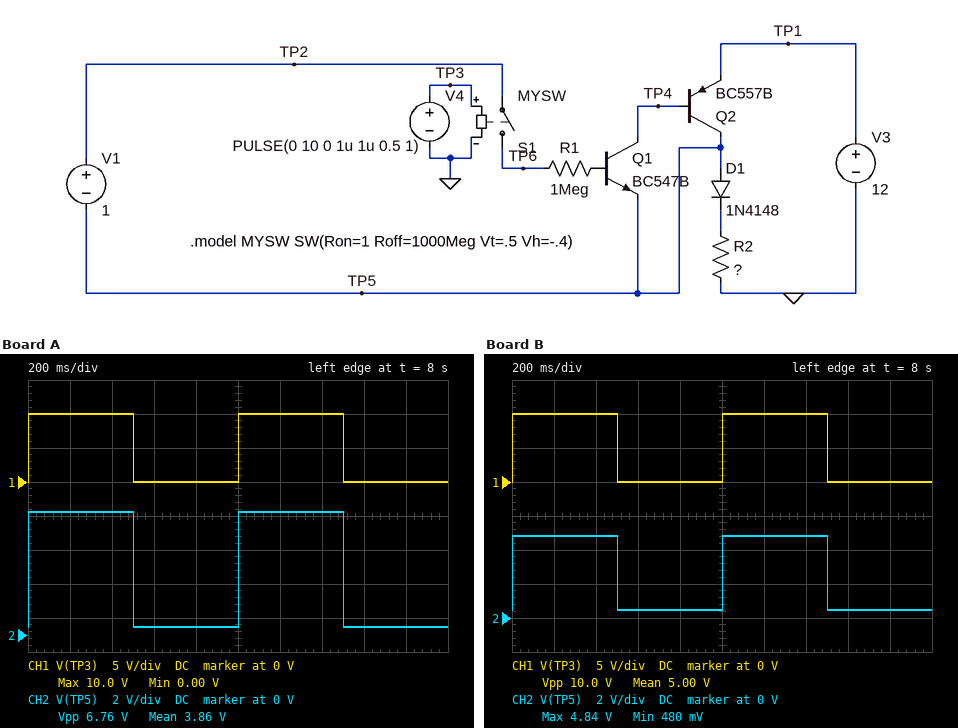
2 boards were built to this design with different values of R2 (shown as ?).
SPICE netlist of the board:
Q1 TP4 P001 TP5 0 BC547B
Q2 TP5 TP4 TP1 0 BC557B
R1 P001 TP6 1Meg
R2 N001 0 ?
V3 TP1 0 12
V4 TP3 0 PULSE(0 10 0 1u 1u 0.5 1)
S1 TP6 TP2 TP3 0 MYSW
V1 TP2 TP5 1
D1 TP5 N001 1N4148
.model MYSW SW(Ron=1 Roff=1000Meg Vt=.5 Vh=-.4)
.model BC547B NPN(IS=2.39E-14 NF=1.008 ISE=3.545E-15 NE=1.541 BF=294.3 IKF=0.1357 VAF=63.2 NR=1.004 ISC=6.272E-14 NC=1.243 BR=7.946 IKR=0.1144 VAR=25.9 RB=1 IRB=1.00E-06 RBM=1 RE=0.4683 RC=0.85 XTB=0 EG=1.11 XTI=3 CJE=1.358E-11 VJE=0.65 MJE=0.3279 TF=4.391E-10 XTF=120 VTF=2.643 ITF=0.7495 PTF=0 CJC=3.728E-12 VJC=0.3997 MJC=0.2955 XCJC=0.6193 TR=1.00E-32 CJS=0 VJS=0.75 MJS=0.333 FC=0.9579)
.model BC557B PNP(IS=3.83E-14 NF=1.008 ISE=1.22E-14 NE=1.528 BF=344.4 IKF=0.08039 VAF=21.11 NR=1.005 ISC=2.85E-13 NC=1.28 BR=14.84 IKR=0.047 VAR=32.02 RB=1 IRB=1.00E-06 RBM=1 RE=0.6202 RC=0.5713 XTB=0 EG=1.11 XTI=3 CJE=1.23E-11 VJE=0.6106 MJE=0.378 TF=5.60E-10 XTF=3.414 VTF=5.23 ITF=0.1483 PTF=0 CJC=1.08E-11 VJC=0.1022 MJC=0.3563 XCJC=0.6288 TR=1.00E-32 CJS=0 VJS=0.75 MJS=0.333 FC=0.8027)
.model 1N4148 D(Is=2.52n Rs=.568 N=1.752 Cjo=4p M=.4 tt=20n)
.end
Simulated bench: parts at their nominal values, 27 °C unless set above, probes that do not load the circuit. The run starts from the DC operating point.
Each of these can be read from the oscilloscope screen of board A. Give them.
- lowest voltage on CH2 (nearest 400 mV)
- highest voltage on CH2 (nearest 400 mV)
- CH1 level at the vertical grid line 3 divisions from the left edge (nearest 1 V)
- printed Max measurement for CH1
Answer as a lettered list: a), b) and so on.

a) 400 mV
b) 7.2 V
c) 0 V
d) 10.0 V
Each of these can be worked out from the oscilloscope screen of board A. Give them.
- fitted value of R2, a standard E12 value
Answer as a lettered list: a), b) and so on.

a) 180 Ω
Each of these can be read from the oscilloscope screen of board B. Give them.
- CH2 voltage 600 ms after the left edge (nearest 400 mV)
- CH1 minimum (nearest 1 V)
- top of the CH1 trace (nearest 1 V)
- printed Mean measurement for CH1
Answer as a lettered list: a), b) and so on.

a) 400 mV
b) 0 V
c) 10 V
d) 5.00 V
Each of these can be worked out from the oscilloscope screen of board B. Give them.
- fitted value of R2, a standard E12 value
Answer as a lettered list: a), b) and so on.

a) 100 Ω
